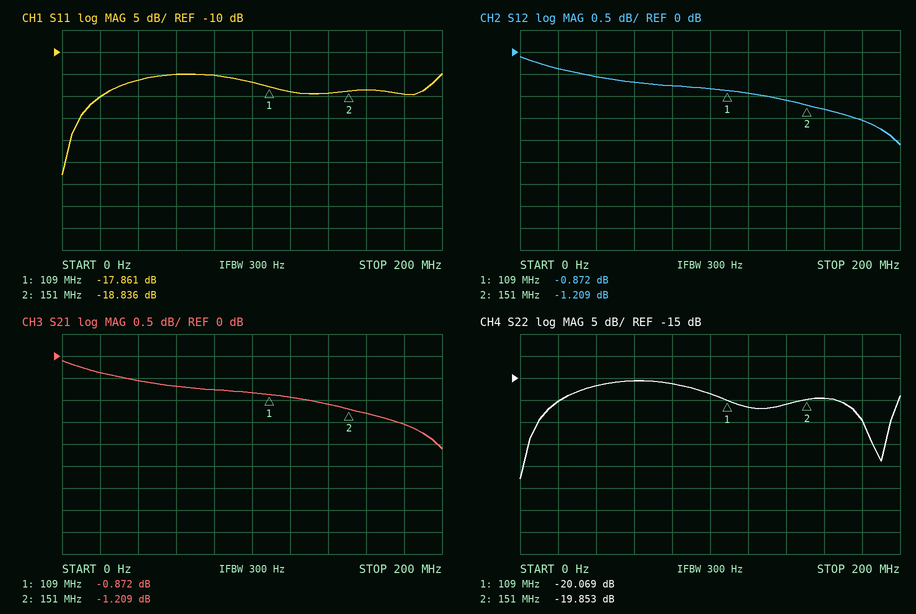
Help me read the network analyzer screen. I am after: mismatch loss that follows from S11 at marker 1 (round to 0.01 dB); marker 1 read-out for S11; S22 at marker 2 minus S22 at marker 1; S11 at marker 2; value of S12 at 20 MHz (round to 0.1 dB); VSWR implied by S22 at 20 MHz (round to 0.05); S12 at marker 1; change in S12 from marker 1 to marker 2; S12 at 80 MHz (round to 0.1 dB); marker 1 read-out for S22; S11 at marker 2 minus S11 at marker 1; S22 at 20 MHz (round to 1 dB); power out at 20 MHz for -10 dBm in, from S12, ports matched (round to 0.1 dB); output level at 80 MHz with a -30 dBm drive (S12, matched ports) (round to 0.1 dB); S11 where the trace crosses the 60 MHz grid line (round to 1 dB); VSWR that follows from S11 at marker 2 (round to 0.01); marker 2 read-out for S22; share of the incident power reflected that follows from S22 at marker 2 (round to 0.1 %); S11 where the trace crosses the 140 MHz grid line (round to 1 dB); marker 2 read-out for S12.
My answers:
0.07 dB
-17.861 dB
0.216 dB
-18.836 dB
-0.4 dB
1.20
-0.872 dB
-0.337 dB
-0.8 dB
-20.069 dB
-0.975 dB
-20 dB
-10.4 dBm
-30.8 dBm
-15 dB
1.26
-19.853 dB
1.0 %
-19 dB
-1.209 dB
